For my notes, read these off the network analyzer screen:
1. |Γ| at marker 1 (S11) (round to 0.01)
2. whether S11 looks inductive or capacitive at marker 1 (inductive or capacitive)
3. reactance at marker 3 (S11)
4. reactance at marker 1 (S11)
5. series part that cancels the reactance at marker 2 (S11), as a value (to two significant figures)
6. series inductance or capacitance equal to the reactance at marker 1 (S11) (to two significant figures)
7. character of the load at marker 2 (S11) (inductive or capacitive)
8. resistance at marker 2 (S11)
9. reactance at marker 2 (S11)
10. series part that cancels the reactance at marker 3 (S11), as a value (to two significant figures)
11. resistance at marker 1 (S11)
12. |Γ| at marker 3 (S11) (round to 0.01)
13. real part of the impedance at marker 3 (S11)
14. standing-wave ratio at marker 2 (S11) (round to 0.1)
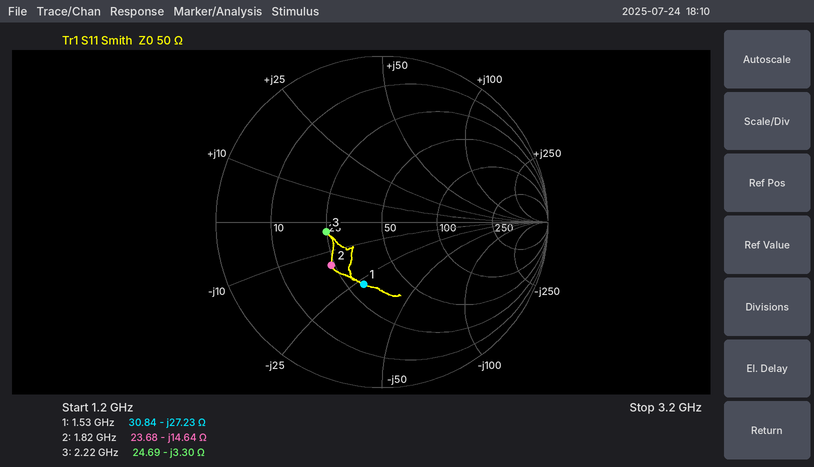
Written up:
0.39
capacitive
-3.30 Ω
-27.23 Ω
1.3 nH
3.8 pF
capacitive
23.68 Ω
-14.64 Ω
240 pH
30.84 Ω
0.34
24.69 Ω
2.3
